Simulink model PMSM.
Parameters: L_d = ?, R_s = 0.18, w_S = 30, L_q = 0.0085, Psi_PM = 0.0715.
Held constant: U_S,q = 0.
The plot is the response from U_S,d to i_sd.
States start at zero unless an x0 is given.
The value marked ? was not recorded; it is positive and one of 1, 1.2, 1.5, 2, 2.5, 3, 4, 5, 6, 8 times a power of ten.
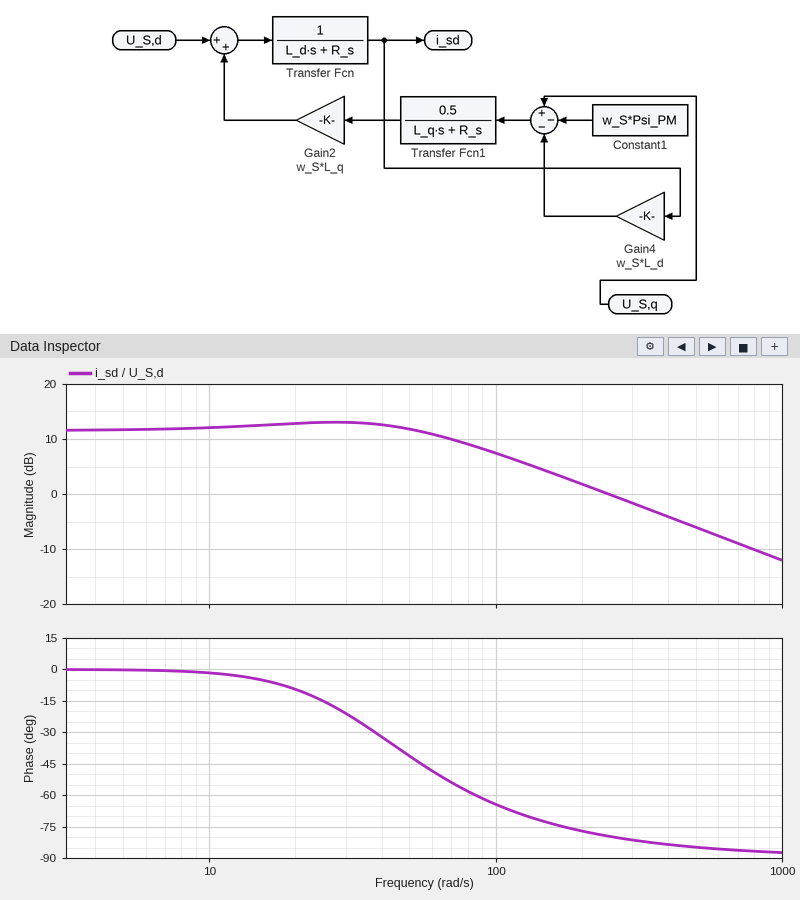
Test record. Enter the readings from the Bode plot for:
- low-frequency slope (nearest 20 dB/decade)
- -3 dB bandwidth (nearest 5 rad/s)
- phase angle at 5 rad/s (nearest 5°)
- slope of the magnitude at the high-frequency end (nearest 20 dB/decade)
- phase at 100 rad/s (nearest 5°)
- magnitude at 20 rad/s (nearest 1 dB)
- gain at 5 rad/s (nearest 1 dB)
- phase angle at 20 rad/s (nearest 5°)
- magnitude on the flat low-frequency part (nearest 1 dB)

0 dB/decade
85 rad/s
0°
-20 dB/decade
-65°
13 dB
12 dB
-10°
12 dB
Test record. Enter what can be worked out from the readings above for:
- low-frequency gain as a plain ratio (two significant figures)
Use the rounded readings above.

4.0
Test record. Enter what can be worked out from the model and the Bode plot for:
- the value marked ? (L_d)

0.004
